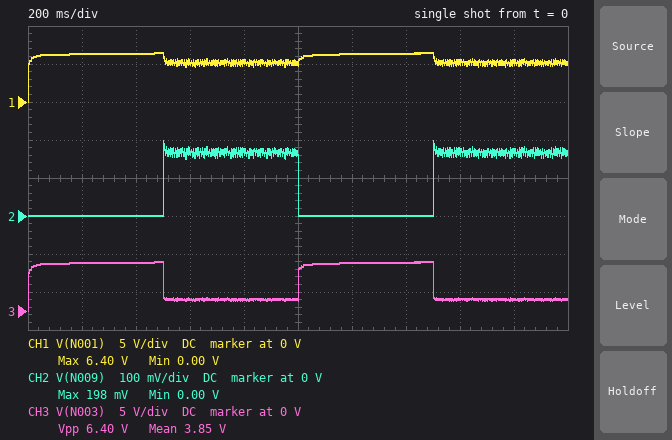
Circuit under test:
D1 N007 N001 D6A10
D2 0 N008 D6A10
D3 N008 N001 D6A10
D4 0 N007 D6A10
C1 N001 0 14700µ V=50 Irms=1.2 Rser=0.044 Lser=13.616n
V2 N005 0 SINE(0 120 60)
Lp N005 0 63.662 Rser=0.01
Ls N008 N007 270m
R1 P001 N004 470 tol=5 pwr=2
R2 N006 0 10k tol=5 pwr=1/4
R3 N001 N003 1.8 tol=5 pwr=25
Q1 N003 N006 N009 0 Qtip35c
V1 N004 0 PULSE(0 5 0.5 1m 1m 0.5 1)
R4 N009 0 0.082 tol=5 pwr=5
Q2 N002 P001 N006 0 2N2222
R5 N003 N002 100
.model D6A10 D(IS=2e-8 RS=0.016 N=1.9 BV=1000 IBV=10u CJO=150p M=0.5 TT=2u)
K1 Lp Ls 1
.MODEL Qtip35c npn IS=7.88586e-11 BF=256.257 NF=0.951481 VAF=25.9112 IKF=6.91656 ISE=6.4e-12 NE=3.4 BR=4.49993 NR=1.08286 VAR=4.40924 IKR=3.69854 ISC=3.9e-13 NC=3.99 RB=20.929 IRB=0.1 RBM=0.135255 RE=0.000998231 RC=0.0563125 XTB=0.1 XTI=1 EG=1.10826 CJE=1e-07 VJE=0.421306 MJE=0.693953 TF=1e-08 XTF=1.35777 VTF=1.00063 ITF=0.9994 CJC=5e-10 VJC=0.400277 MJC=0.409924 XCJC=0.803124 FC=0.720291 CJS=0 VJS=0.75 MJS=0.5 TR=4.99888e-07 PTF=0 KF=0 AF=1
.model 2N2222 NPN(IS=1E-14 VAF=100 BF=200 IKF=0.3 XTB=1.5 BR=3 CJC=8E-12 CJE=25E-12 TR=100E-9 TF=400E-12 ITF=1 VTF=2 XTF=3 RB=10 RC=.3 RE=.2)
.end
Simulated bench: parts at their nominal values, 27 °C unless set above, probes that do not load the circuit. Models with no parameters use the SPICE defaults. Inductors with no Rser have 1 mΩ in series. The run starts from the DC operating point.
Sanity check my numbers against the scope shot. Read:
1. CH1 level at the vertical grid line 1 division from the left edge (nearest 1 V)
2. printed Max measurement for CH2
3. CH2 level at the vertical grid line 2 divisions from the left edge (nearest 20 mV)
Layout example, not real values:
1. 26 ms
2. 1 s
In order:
1. 6 V
2. 198 mV
3. 0 V
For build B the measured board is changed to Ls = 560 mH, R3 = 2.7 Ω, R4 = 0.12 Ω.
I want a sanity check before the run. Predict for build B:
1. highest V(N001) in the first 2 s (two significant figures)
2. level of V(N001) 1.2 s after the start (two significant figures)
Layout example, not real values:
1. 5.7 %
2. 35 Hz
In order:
1. 9.8 V
2. 9.7 V
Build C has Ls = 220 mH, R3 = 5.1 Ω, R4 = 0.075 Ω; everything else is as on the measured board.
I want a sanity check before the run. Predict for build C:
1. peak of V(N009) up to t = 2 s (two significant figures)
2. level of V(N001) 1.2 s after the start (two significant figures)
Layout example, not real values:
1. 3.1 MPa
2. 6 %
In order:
1. 74 mV
2. 5.5 V
